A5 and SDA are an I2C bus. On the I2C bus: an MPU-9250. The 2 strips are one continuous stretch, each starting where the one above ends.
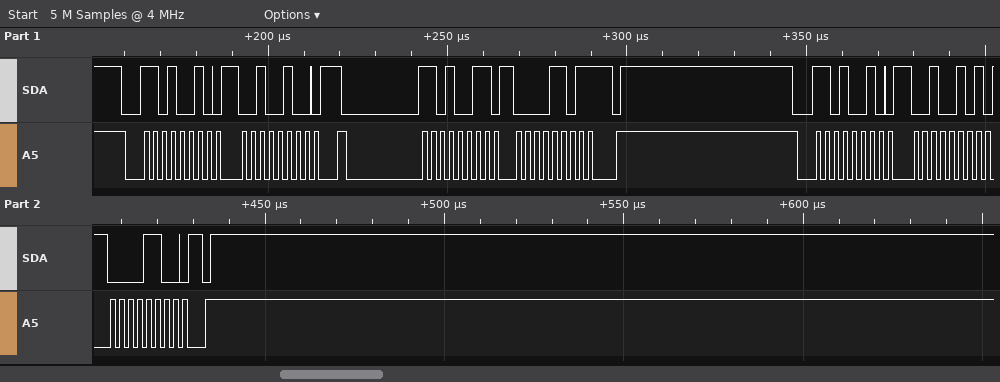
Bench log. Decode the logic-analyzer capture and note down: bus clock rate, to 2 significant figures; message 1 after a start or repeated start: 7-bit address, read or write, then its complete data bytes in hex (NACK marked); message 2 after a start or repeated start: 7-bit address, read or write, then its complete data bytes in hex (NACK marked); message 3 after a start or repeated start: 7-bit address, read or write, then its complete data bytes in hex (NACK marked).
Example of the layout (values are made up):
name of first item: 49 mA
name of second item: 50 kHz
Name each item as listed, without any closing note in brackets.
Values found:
bus clock rate, to 2 significant figures: 400 kHz
message 1 after a start or repeated start: 7-bit address, read or write, then its complete data bytes in hex: 0x69 write: 24
message 2 after a start or repeated start: 7-bit address, read or write, then its complete data bytes in hex: 0x69 read: 0D NACK
message 3 after a start or repeated start: 7-bit address, read or write, then its complete data bytes in hex: 0x69 write: 25 0C
